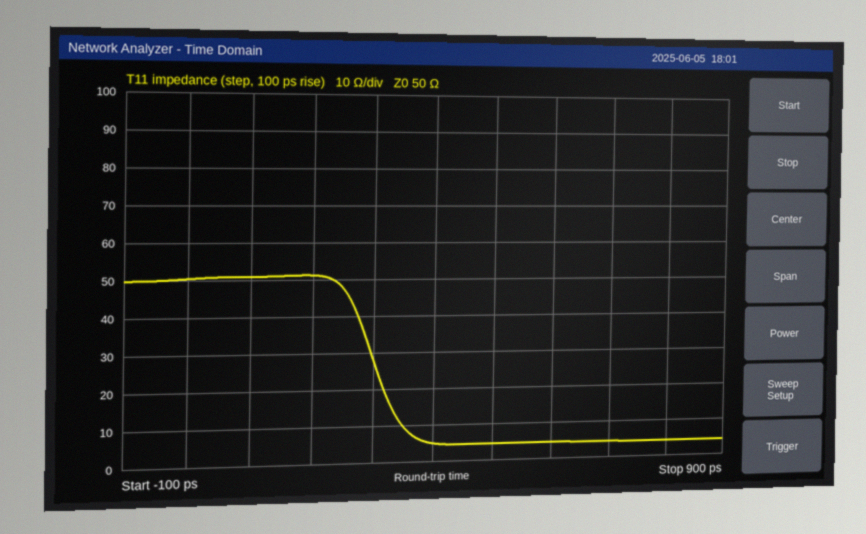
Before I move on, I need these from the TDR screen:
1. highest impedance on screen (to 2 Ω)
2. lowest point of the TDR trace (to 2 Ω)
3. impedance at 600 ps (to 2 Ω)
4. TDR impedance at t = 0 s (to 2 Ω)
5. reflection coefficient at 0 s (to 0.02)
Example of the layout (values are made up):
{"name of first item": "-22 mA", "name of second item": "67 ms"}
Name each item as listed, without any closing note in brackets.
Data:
{"highest impedance on screen": "52 Ω", "lowest point of the TDR trace": "4 Ω", "impedance at 600 ps": "4 Ω", "TDR impedance at t = 0 s": "50 Ω", "reflection coefficient at 0 s": "0.00"}
